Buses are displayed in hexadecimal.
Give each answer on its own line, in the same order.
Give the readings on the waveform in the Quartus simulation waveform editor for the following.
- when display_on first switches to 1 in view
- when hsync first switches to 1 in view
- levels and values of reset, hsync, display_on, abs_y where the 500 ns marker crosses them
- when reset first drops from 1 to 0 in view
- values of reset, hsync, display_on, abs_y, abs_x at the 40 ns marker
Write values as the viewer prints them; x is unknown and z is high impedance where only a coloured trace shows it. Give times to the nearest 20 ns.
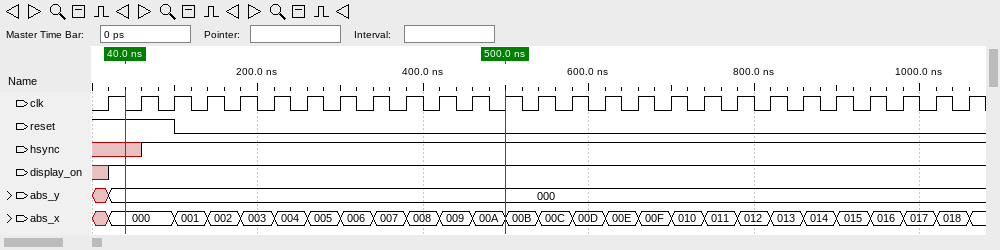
20 ns
60 ns
reset=0, hsync=1, display_on=1, abs_y=000
100 ns
reset=1, hsync=x, display_on=1, abs_y=000, abs_x=000
